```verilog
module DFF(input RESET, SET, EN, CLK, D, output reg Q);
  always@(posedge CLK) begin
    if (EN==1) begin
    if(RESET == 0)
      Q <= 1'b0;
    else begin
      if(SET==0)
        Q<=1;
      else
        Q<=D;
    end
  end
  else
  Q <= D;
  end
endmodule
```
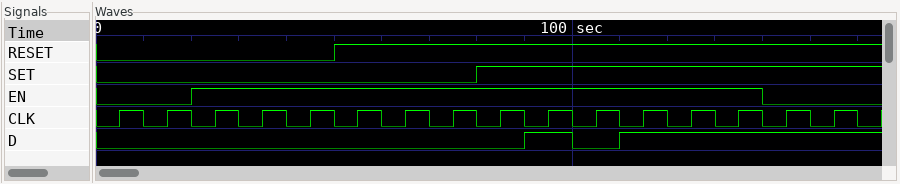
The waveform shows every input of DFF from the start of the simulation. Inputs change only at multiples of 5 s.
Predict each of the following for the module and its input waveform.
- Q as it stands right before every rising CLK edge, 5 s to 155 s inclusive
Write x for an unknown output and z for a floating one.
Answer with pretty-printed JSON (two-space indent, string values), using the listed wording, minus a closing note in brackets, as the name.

{
  "Q as it stands right before every rising CLK edge, 5 s to 155 s inclusive": "x 0 0 0 0 0 1 1 1 0 1 0 1 1 1 1"
}
